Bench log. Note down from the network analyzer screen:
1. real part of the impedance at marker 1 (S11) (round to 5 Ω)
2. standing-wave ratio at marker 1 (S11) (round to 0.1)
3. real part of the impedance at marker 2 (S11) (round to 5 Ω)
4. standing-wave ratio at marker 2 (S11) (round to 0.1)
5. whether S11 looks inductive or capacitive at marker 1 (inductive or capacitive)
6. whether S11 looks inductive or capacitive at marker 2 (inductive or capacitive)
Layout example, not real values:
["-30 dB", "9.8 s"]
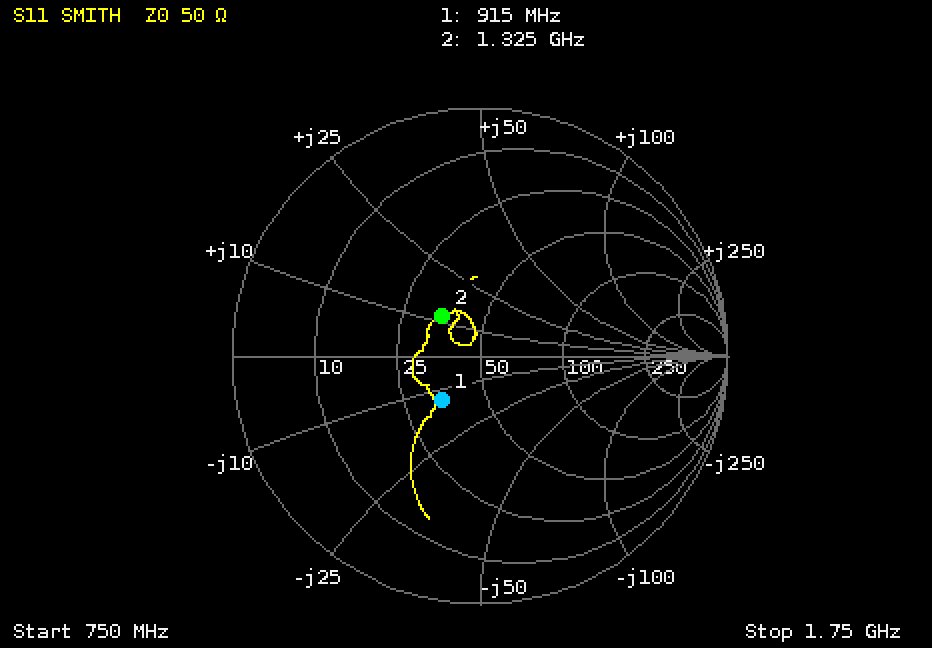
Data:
["35 Ω", "1.6", "35 Ω", "1.6", "capacitive", "inductive"]
